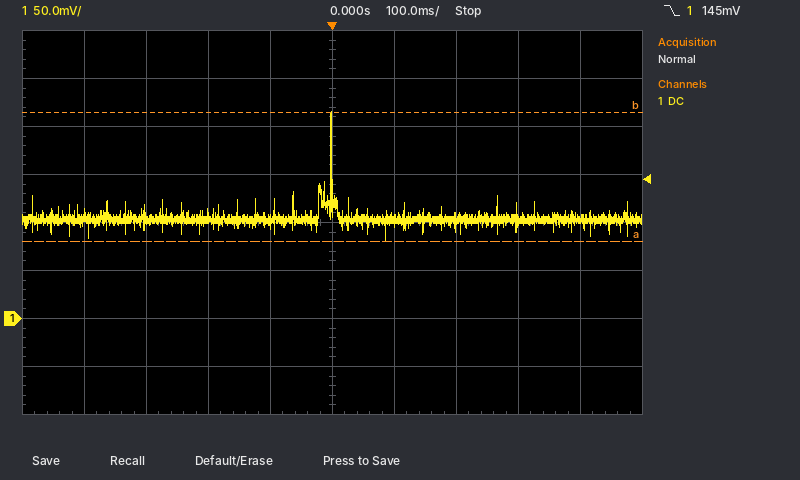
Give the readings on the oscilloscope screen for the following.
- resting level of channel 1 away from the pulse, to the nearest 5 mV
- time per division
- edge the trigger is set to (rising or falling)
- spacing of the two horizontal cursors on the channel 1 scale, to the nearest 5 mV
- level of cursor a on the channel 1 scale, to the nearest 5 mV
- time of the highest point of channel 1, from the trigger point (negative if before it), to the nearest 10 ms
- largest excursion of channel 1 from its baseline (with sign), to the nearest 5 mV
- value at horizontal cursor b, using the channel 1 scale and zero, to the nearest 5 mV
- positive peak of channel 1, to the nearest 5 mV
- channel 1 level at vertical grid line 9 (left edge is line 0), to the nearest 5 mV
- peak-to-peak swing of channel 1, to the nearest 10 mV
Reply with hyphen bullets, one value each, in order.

- 105 mV
- 100 ms
- falling
- 135 mV
- 80 mV
- 0 ms
- +110 mV
- 215 mV
- 215 mV
- 105 mV
- 130 mV
